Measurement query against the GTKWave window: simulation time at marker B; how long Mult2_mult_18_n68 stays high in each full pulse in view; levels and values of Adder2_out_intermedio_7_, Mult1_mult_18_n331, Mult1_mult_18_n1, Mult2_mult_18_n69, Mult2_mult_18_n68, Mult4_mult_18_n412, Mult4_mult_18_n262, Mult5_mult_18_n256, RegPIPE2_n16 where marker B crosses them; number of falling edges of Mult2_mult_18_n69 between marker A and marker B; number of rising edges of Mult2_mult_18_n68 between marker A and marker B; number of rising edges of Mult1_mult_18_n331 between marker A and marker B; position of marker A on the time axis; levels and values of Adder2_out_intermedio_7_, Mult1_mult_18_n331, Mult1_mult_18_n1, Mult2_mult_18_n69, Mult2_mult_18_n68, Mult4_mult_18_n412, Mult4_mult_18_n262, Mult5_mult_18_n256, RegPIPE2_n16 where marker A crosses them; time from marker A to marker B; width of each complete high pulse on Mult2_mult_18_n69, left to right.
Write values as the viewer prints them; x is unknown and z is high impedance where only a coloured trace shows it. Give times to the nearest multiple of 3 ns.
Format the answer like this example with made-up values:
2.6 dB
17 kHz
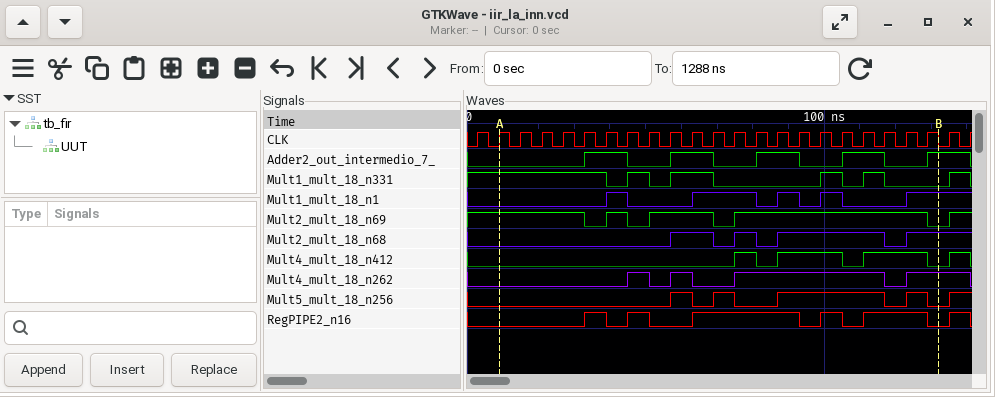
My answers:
132 ns
12 ns, 6 ns, 30 ns
Adder2_out_intermedio_7_=1, Mult1_mult_18_n331=0, Mult1_mult_18_n1=1, Mult2_mult_18_n69=0, Mult2_mult_18_n68=1, Mult4_mult_18_n412=0, Mult4_mult_18_n262=1, Mult5_mult_18_n256=0, RegPIPE2_n16=0
4
4
4
9 ns
Adder2_out_intermedio_7_=0, Mult1_mult_18_n331=1, Mult1_mult_18_n1=0, Mult2_mult_18_n69=1, Mult2_mult_18_n68=0, Mult4_mult_18_n412=0, Mult4_mult_18_n262=0, Mult5_mult_18_n256=0, RegPIPE2_n16=0
123 ns
6 ns, 18 ns, 54 ns
